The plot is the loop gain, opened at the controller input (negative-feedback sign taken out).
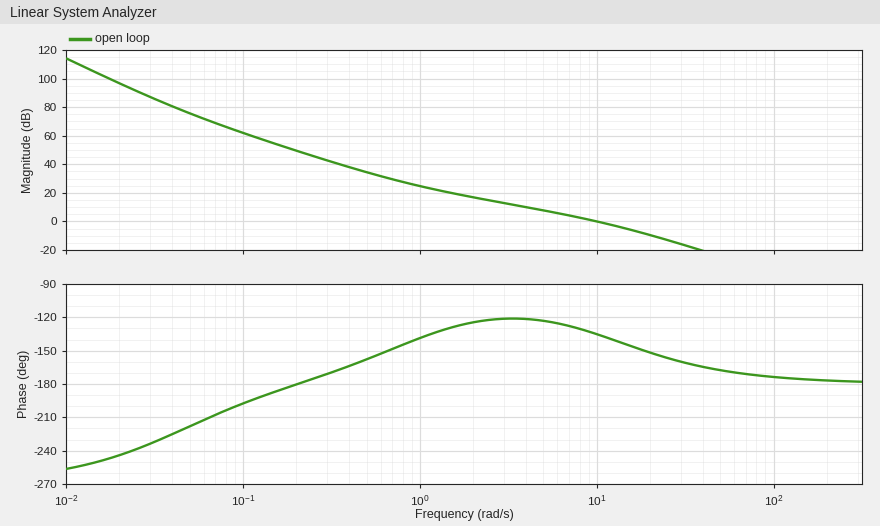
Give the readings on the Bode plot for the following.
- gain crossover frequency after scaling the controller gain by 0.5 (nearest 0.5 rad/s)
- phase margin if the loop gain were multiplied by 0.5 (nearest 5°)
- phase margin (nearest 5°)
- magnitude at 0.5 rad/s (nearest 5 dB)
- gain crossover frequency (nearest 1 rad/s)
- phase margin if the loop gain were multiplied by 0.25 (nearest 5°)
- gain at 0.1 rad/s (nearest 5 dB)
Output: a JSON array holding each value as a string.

["6.0 rad/s", "55°", "45°", "35 dB", "10 rad/s", "60°", "60 dB"]
